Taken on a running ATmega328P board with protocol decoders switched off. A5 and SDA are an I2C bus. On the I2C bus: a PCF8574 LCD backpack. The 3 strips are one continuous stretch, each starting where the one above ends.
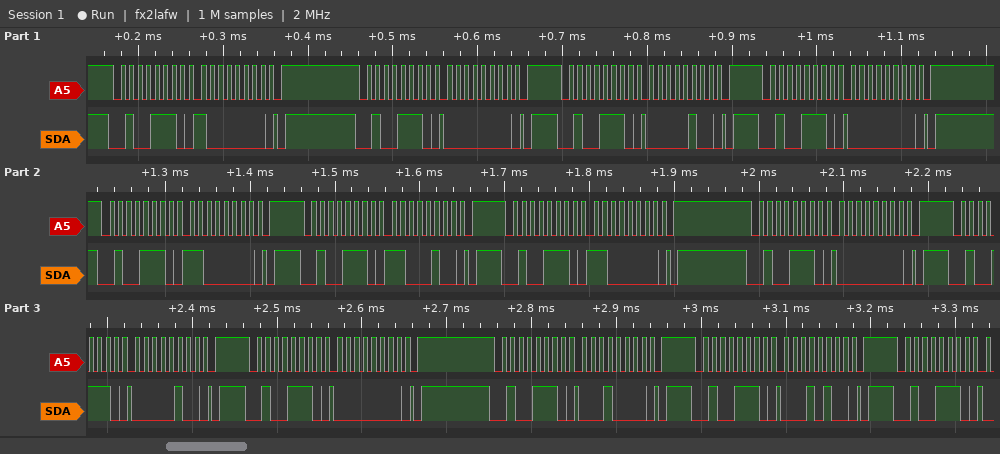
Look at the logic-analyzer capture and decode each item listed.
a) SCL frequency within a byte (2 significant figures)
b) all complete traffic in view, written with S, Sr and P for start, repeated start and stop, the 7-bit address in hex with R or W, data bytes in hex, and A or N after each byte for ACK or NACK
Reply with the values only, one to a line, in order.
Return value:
100 kHz
S 27W A 80 A P S 27W A 00 A P S 27W A 04 A P S 27W A 00 A P S 27W A C0 A P S 27W A C4 A P S 27W A C0 A P S 27W A 00 A P S 27W A 04 A P S 27W A 00 A P S 27W A 10 A P S 27W A 14 A P S 27W A
